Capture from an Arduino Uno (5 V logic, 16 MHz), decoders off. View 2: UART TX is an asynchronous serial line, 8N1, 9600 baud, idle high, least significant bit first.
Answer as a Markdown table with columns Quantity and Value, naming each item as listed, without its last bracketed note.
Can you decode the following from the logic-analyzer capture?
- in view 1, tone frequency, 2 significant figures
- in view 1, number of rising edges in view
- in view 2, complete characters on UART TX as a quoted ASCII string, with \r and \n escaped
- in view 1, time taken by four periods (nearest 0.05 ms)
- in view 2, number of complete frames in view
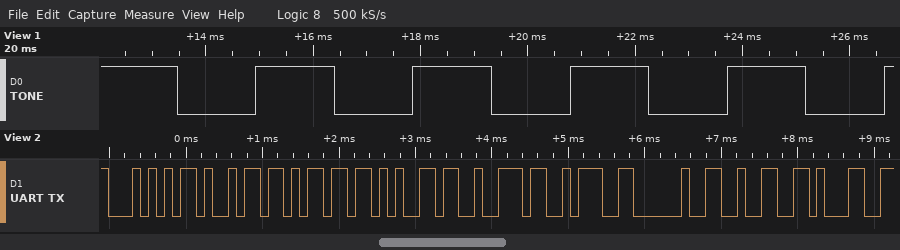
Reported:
| Quantity | Value |
|---|---|
| in view 1, tone frequency, 2 significant figures | 340 Hz |
| in view 1, number of rising edges in view | 5 |
| in view 2, complete characters on UART TX as a quoted ASCII string, with \r and \n escaped | "Timer: 21" |
| in view 1, time taken by four periods | 11.70 ms |
| in view 2, number of complete frames in view | 9 |
